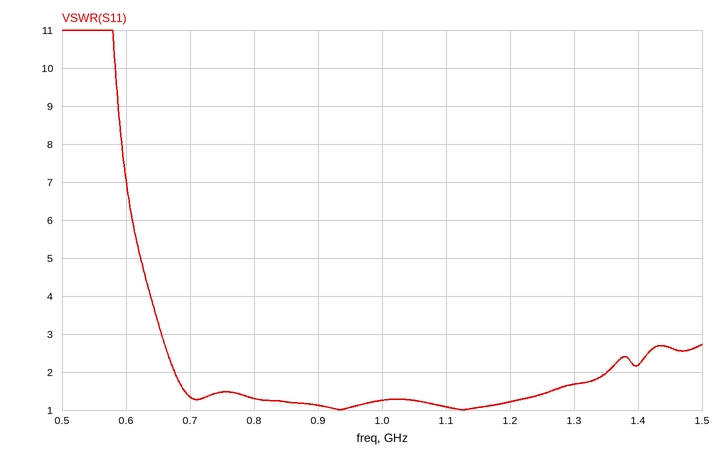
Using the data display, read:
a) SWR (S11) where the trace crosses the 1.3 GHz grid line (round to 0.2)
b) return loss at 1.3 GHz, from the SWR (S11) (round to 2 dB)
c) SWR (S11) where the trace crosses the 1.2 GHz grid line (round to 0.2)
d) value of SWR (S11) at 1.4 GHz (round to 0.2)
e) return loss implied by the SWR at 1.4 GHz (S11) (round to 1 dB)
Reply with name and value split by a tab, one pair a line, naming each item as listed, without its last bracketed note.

SWR (S11) where the trace crosses the 1.3 GHz grid line	1.6
return loss at 1.3 GHz, from the SWR (S11)	12 dB
SWR (S11) where the trace crosses the 1.2 GHz grid line	1.2
value of SWR (S11) at 1.4 GHz	2.2
return loss implied by the SWR at 1.4 GHz (S11)	9 dB
